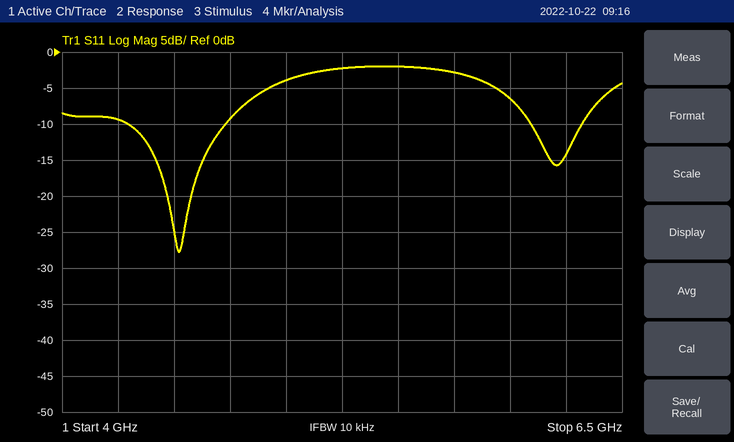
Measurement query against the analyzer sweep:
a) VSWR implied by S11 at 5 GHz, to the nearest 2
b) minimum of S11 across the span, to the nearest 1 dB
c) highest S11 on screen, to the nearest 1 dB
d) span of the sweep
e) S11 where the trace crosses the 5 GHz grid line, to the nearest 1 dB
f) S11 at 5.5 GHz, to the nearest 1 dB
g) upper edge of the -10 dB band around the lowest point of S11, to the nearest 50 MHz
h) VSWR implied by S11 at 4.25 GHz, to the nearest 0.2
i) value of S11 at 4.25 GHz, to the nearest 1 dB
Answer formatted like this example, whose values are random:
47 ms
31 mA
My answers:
4
-28 dB
-2 dB
2.5 GHz
-4 dB
-2 dB
4.75 GHz
2.0
-9 dB
